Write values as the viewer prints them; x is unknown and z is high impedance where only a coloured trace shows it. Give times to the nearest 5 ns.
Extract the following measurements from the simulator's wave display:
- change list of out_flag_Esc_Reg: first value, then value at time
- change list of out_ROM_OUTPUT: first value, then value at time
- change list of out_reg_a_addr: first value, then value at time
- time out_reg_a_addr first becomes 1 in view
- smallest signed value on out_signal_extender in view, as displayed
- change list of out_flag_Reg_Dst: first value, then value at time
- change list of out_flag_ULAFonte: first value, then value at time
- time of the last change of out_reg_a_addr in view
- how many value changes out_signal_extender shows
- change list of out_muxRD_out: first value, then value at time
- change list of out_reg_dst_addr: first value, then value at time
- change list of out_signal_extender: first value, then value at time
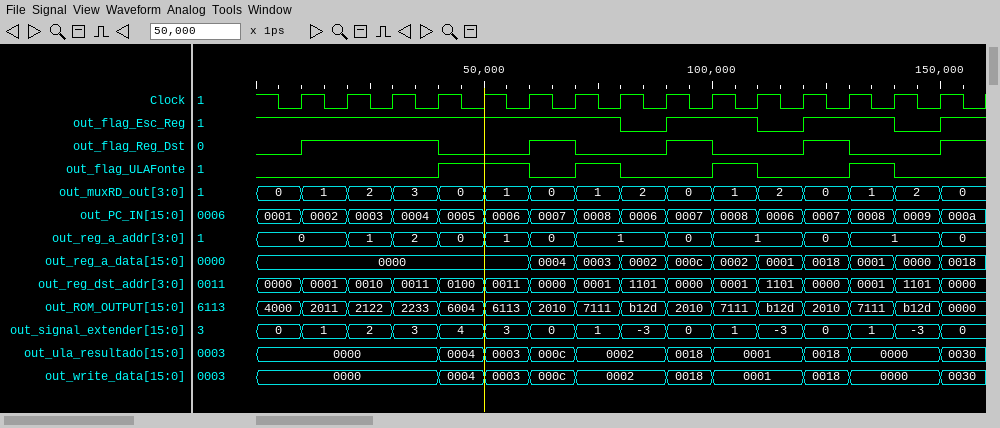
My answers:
1, 0 at 80 ns, 1 at 90 ns, 0 at 110 ns, 1 at 120 ns, 0 at 140 ns, 1 at 150 ns
4000, 2011 at 10 ns, 2122 at 20 ns, 2233 at 30 ns, 6004 at 40 ns, 6113 at 50 ns, 2010 at 60 ns, 7111 at 70 ns, b12d at 80 ns, 2010 at 90 ns, 7111 at 100 ns, b12d at 110 ns, 2010 at 120 ns, 7111 at 130 ns, b12d at 140 ns, 0000 at 150 ns
0, 1 at 20 ns, 2 at 30 ns, 0 at 40 ns, 1 at 50 ns, 0 at 60 ns, 1 at 70 ns, 0 at 90 ns, 1 at 100 ns, 0 at 120 ns, 1 at 130 ns, 0 at 150 ns
20 ns
-3
0, 1 at 10 ns, 0 at 40 ns, 1 at 60 ns, 0 at 70 ns, 1 at 90 ns, 0 at 100 ns, 1 at 120 ns, 0 at 130 ns, 1 at 150 ns
0, 1 at 40 ns, 0 at 60 ns, 1 at 70 ns, 0 at 80 ns, 1 at 100 ns, 0 at 110 ns, 1 at 130 ns, 0 at 140 ns
150 ns
15
0, 1 at 10 ns, 2 at 20 ns, 3 at 30 ns, 0 at 40 ns, 1 at 50 ns, 0 at 60 ns, 1 at 70 ns, 2 at 80 ns, 0 at 90 ns, 1 at 100 ns, 2 at 110 ns, 0 at 120 ns, 1 at 130 ns, 2 at 140 ns, 0 at 150 ns
0000, 0001 at 10 ns, 0010 at 20 ns, 0011 at 30 ns, 0100 at 40 ns, 0011 at 50 ns, 0000 at 60 ns, 0001 at 70 ns, 1101 at 80 ns, 0000 at 90 ns, 0001 at 100 ns, 1101 at 110 ns, 0000 at 120 ns, 0001 at 130 ns, 1101 at 140 ns, 0000 at 150 ns
0, 1 at 10 ns, 2 at 20 ns, 3 at 30 ns, 4 at 40 ns, 3 at 50 ns, 0 at 60 ns, 1 at 70 ns, -3 at 80 ns, 0 at 90 ns, 1 at 100 ns, -3 at 110 ns, 0 at 120 ns, 1 at 130 ns, -3 at 140 ns, 0 at 150 ns
